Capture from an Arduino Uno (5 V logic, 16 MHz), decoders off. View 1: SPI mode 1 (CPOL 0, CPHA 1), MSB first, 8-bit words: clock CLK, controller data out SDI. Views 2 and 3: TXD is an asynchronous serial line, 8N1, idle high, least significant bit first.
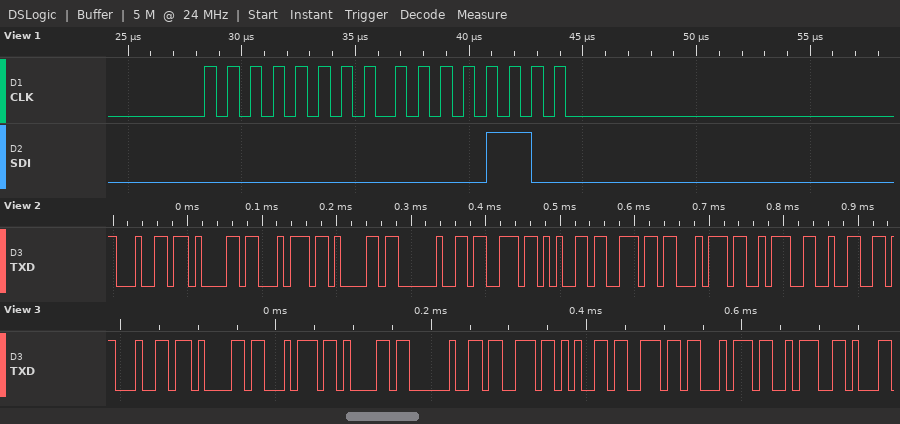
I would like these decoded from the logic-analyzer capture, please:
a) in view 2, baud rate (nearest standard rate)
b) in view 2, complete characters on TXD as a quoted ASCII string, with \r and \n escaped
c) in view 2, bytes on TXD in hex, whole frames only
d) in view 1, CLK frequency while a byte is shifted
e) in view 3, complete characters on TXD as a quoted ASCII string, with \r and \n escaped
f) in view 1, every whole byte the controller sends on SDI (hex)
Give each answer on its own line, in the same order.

115200 baud
"data sent:2"
0x64 0x61 0x74 0x61 0x20 0x73 0x65 0x6E 0x74 0x3A 0x32
1 MHz
"data sent:"
0x00 0x0C
